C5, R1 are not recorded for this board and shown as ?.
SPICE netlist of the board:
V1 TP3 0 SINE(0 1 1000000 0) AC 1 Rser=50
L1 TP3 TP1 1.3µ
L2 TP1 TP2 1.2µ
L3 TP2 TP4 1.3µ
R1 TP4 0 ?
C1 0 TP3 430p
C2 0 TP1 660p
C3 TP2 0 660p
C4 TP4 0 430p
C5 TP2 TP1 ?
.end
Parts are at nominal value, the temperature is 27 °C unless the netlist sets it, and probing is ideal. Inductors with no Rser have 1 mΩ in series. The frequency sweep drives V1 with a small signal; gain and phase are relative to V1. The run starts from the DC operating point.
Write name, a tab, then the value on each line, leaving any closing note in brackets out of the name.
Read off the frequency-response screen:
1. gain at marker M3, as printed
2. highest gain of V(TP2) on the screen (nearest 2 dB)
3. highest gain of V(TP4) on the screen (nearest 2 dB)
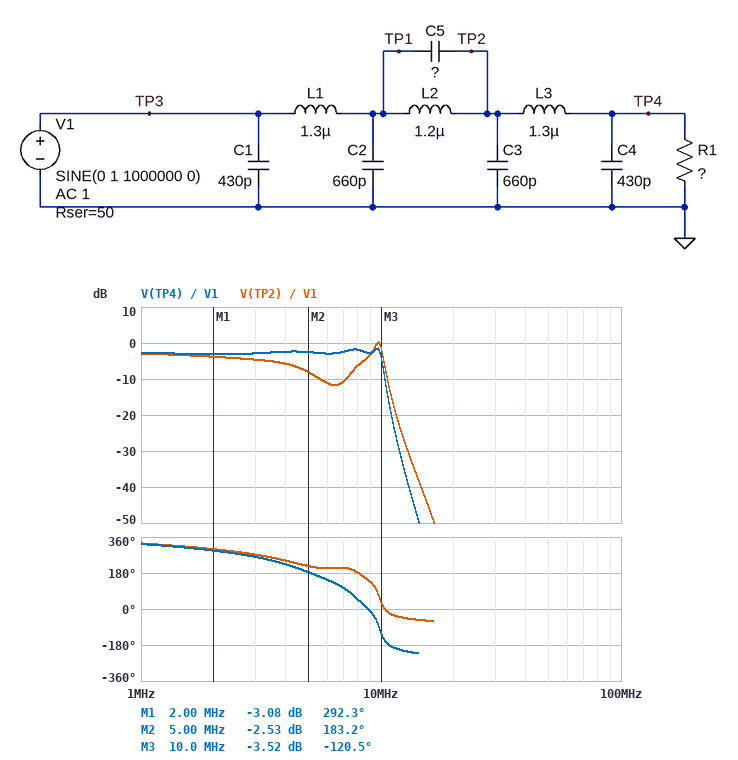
gain at marker M3, as printed	-3.52 dB
highest gain of V(TP2) on the screen	0 dB
highest gain of V(TP4) on the screen	-2 dB
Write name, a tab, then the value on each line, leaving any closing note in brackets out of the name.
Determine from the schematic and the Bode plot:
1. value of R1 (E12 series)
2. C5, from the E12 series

value of R1	150 Ω
C5, from the E12 series	47 pF
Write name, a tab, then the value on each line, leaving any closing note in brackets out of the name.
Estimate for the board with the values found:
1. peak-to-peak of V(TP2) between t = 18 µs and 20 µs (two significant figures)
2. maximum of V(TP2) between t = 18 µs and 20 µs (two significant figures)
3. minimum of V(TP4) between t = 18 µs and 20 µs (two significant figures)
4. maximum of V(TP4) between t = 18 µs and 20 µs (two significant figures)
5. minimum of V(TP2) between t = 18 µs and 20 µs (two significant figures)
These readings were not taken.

peak-to-peak of V(TP2) between t = 18 µs and 20 µs	1.4 V
maximum of V(TP2) between t = 18 µs and 20 µs	710 mV
minimum of V(TP4) between t = 18 µs and 20 µs	-730 mV
maximum of V(TP4) between t = 18 µs and 20 µs	730 mV
minimum of V(TP2) between t = 18 µs and 20 µs	-710 mV
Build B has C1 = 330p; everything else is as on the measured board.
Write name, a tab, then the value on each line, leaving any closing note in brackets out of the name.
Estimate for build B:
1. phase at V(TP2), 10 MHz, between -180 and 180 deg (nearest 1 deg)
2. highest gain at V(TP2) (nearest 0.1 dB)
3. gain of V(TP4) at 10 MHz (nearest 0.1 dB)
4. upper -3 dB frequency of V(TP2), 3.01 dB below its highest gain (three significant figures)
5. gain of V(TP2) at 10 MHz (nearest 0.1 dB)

phase at V(TP2), 10 MHz, between -180 and 180 deg	50 deg
highest gain at V(TP2)	0.2 dB
gain of V(TP4) at 10 MHz	-3.7 dB
upper -3 dB frequency of V(TP2), 3.01 dB below its highest gain	10.1 MHz
gain of V(TP2) at 10 MHz	-1.3 dB
